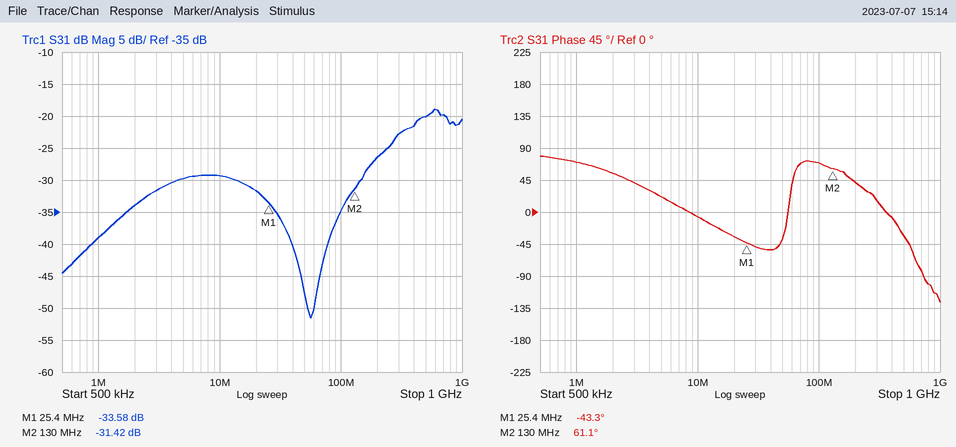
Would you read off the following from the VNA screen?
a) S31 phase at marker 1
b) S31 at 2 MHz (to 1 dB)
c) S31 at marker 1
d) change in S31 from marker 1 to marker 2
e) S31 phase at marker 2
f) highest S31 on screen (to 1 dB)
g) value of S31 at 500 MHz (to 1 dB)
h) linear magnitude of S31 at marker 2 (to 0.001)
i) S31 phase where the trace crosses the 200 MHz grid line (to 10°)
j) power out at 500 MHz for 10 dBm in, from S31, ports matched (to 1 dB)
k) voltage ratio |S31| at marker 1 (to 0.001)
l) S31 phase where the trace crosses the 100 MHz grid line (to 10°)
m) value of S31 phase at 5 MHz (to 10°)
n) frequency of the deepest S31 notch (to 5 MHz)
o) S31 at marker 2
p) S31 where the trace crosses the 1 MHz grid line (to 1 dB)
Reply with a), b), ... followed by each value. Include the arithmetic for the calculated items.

a) -43.3°
b) -34 dB
c) -33.58 dB
d) -31.42 − (-33.58) = 2.16 dB
e) 61.1°
f) -19 dB
g) -20 dB
h) 10^(-31.42/20) ≈ 0.027
i) 40°
j) 10 dBm + (-20 dB) = -10 dBm
k) 10^(-33.58/20) ≈ 0.021
l) 70°
m) 20°
n) 55 MHz
o) -31.42 dB
p) -39 dB
